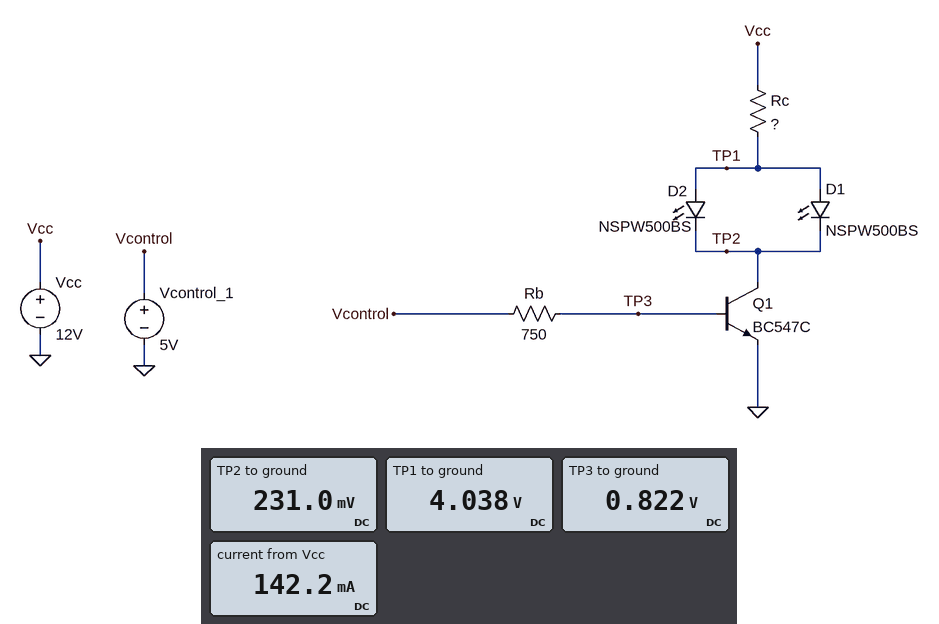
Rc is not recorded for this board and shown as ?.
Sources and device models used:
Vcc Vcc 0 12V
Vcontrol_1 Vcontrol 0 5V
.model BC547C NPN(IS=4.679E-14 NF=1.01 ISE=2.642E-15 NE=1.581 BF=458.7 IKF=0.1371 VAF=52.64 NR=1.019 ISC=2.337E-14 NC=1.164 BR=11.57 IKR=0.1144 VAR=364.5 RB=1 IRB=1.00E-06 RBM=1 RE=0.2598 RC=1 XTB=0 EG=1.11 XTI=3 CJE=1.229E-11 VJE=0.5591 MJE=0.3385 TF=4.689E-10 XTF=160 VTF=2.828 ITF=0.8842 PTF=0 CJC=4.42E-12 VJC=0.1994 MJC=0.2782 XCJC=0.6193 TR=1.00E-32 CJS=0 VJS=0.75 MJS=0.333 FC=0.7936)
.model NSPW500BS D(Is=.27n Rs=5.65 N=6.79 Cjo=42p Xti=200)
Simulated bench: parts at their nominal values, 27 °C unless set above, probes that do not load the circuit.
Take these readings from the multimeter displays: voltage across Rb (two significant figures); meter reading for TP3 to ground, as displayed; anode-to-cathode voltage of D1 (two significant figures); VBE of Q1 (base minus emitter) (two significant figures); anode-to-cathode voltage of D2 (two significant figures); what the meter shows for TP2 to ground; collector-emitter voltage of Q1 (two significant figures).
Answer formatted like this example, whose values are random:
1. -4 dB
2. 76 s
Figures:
1. 4.2 V
2. 0.822 V
3. 3.8 V
4. 820 mV
5. 3.8 V
6. 231.0 mV
7. 230 mV
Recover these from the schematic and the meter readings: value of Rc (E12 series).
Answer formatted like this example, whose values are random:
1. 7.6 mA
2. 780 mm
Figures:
1. 56 Ω
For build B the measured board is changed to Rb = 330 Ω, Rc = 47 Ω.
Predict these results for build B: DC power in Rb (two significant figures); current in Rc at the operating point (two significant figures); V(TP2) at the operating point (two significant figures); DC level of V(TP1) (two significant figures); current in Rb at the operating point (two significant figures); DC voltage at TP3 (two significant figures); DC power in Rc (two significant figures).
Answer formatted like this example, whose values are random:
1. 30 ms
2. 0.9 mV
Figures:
1. 52 mW
2. 170 mA
3. 250 mV
4. 4.2 V
5. 13 mA
6. 850 mV
7. 1.3 W
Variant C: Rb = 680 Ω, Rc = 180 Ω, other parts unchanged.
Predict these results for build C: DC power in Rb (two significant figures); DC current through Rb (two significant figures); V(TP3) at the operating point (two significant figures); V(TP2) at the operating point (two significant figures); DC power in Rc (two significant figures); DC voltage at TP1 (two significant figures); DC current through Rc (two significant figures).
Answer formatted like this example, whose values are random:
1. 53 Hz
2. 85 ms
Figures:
1. 26 mW
2. 6.2 mA
3. 770 mV
4. 82 mV
5. 410 mW
6. 3.4 V
7. 48 mA
